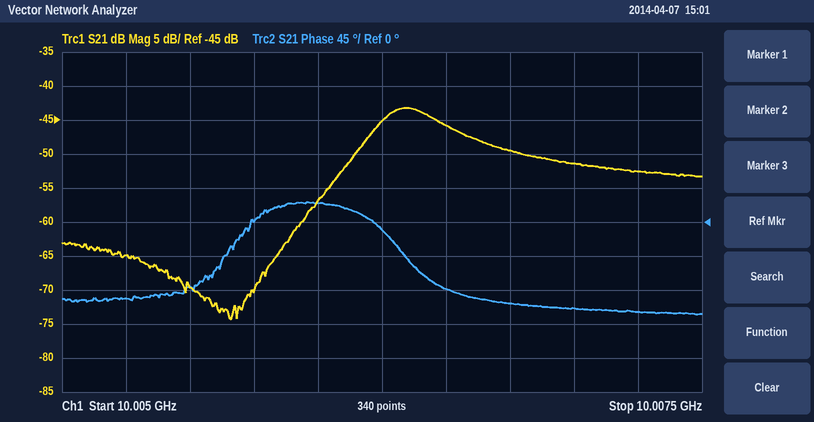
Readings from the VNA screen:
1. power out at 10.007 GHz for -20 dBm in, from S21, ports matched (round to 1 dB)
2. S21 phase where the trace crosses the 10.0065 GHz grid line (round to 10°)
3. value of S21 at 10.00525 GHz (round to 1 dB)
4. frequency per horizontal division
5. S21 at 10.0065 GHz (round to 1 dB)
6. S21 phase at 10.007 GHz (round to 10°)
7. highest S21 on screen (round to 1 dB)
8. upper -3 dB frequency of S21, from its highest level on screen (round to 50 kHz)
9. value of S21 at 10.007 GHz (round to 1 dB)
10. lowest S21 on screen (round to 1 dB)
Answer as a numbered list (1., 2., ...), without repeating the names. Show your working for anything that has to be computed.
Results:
1. -20 dBm + (-51 dB) = -71 dBm
2. -90°
3. -65 dB
4. 250 kHz
5. -46 dB
6. -110°
7. -43 dB
8. 10.00650 GHz
9. -51 dB
10. -74 dB
